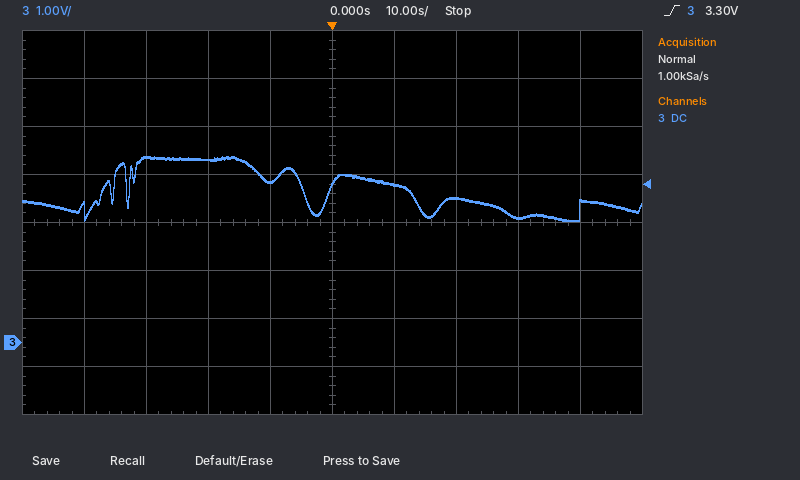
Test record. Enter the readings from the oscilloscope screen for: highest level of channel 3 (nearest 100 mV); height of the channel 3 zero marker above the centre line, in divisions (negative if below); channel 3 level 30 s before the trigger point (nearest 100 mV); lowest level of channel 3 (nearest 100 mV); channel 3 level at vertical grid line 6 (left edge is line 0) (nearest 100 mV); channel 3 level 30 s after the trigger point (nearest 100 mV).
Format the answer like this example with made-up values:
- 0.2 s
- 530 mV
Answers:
- 3.9 V
- -2.5 div
- 3.9 V
- 2.5 V
- 3.3 V
- 2.6 V
